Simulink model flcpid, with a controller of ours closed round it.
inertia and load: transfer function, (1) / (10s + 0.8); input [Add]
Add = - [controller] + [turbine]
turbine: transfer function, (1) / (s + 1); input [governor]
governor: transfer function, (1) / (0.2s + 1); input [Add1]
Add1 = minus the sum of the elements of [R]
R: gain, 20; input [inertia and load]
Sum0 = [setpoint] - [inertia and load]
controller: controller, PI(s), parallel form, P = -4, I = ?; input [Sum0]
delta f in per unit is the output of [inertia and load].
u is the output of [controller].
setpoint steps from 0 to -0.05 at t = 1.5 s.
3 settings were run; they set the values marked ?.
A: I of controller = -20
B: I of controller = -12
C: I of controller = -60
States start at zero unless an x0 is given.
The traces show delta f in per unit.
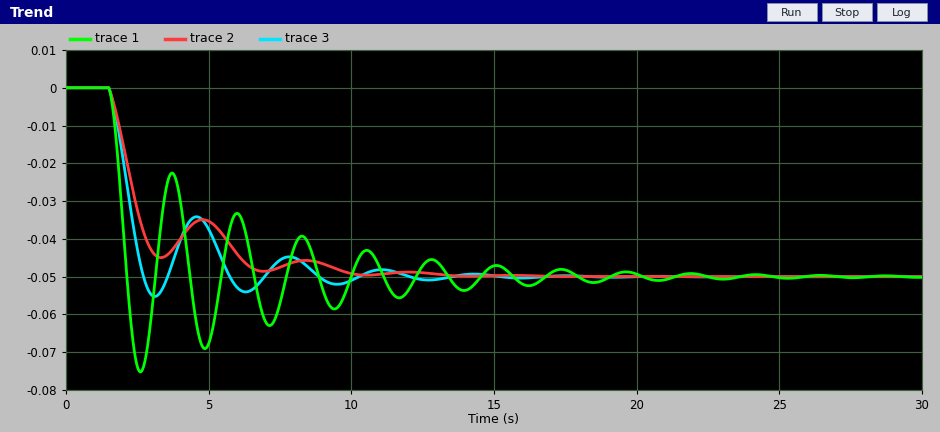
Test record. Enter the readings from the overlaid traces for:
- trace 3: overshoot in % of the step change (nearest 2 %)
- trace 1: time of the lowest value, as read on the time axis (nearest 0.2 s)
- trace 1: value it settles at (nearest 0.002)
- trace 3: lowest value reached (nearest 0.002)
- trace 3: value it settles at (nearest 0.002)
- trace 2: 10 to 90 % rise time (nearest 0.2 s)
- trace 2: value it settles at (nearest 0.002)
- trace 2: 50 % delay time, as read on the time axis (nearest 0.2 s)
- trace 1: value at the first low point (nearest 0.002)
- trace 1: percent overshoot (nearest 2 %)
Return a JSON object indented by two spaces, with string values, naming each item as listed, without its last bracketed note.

{
  "trace 3: overshoot in % of the step change": "10 %",
  "trace 1: time of the lowest value, as read on the time axis": "2.6 s",
  "trace 1: value it settles at": "-0.050",
  "trace 3: lowest value reached": "-0.056",
  "trace 3: value it settles at": "-0.050",
  "trace 2: 10 to 90 % rise time": "4.4 s",
  "trace 2: value it settles at": "-0.050",
  "trace 2: 50 % delay time, as read on the time axis": "2.2 s",
  "trace 1: value at the first low point": "-0.076",
  "trace 1: percent overshoot": "50 %"
}
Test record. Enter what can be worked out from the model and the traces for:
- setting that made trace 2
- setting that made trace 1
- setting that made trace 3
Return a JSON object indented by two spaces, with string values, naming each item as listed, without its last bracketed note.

{
  "setting that made trace 2": "B",
  "setting that made trace 1": "C",
  "setting that made trace 3": "A"
}
